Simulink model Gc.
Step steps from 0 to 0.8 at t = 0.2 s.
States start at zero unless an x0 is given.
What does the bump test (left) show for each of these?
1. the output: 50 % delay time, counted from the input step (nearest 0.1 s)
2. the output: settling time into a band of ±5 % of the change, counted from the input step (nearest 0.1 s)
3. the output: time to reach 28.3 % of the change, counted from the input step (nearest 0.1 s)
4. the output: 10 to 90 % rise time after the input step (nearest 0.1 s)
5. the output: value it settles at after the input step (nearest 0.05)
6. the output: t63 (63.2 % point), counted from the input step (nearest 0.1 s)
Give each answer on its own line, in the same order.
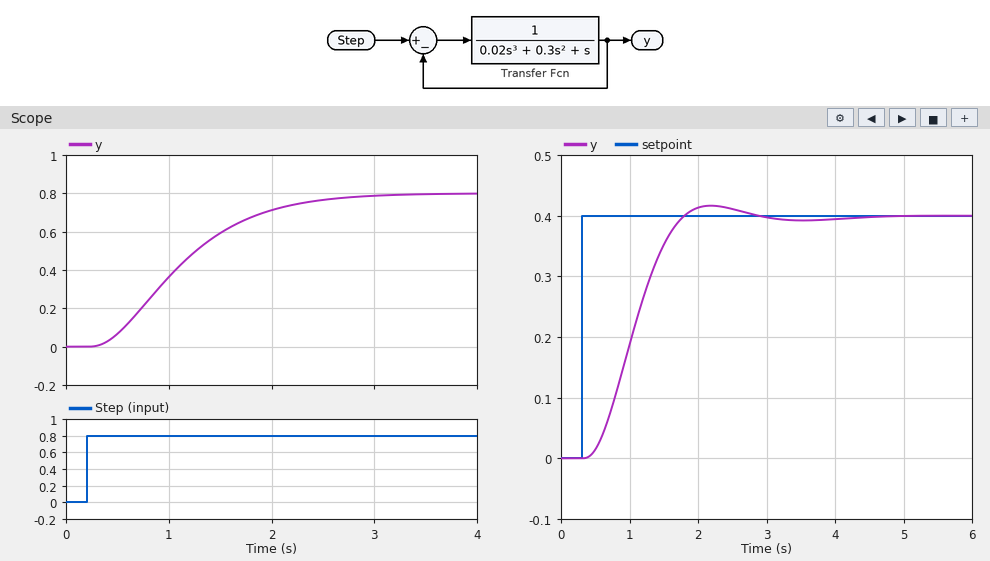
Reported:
0.9 s
2.2 s
0.6 s
1.5 s
0.80
1.1 s
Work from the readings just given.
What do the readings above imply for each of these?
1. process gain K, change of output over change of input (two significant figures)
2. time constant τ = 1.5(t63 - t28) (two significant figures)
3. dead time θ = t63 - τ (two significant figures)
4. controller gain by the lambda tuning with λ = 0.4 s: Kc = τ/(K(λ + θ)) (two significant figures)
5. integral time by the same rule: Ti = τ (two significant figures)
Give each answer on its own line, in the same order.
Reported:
1.0
0.75 s
0.35 s
1.0
0.75 s
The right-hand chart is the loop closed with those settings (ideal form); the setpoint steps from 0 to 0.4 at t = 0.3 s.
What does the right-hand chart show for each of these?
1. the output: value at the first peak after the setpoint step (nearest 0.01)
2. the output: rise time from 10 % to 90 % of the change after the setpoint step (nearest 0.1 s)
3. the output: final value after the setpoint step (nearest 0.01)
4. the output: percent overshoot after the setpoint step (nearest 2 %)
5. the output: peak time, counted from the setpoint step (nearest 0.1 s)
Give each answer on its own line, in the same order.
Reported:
0.42
0.9 s
0.40
4 %
1.9 s
